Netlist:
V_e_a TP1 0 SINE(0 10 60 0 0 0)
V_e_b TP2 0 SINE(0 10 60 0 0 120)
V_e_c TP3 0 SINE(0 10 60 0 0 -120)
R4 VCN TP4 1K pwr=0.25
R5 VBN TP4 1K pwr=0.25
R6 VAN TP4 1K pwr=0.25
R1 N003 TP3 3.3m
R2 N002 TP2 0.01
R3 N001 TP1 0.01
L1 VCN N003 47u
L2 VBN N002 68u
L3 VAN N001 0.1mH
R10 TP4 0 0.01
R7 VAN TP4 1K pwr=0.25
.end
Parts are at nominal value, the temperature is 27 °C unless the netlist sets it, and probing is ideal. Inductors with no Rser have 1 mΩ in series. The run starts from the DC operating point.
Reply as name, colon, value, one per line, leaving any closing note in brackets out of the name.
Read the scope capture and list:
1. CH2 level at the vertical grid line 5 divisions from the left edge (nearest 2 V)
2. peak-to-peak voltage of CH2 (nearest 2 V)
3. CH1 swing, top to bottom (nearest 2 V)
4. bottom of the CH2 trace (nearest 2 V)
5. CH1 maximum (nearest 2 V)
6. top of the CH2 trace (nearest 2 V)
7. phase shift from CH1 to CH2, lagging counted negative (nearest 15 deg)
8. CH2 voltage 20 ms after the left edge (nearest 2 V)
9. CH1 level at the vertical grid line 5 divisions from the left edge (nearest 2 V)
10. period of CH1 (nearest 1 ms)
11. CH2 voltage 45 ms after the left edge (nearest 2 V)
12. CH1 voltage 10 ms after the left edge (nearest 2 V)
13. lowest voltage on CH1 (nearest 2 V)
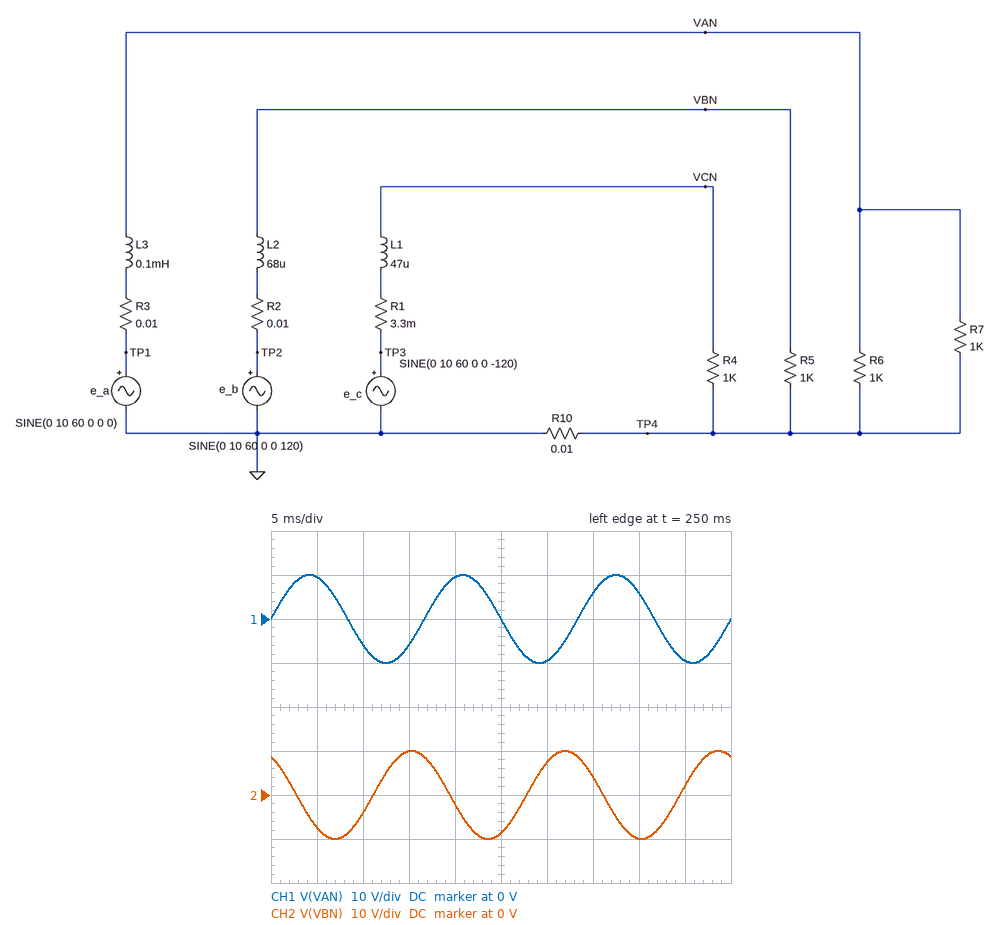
CH2 level at the vertical grid line 5 divisions from the left edge: -8 V
peak-to-peak voltage of CH2: 20 V
CH1 swing, top to bottom: 20 V
bottom of the CH2 trace: -10 V
CH1 maximum: 10 V
top of the CH2 trace: 10 V
phase shift from CH1 to CH2, lagging counted negative: 120 deg
CH2 voltage 20 ms after the left edge: -2 V
CH1 level at the vertical grid line 5 divisions from the left edge: 0 V
period of CH1: 17 ms
CH2 voltage 45 ms after the left edge: 2 V
CH1 voltage 10 ms after the left edge: -6 V
lowest voltage on CH1: -10 V
